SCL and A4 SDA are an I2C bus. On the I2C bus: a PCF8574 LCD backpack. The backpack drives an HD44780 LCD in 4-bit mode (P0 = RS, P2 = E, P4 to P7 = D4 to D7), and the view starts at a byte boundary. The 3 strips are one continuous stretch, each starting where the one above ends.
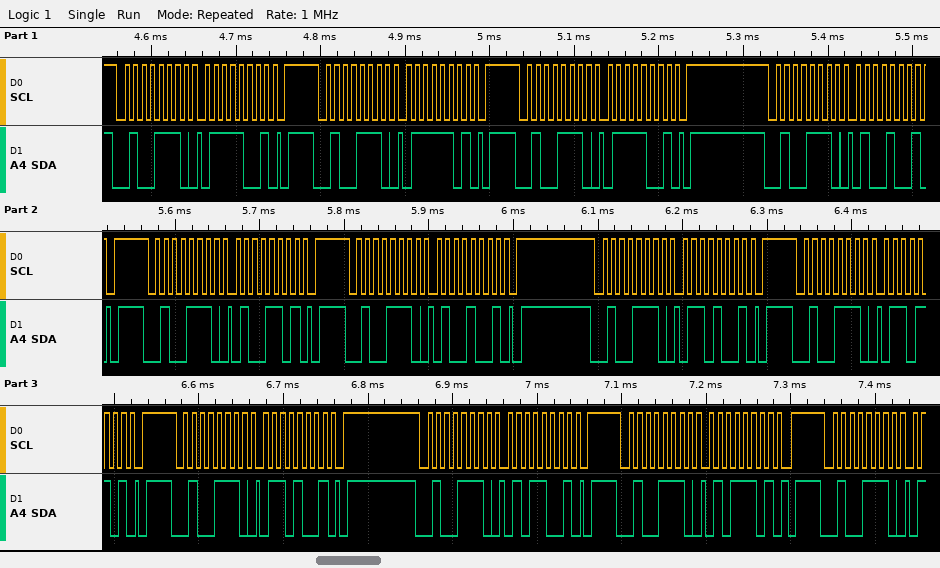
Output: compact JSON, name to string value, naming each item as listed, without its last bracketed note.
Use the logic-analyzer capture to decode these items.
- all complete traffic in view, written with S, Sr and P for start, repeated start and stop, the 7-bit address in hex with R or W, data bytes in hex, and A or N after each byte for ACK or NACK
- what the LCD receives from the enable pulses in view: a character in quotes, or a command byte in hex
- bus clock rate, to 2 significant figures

{"all complete traffic in view, written with S, Sr and P for start, repeated start and stop, the 7-bit address in hex with R or W, data bytes in hex, and A or N after each byte for ACK or NACK": "S 27W A 79 A P S 27W A 7D A P S 27W A 79 A P S 27W A 49 A P S 27W A 4D A P S 27W A 49 A P S 27W A 69 A P S 27W A 6D A P S 27W A 69 A P S 27W A 59 A P S 27W A 5D A P S 27W A", "what the LCD receives from the enable pulses in view: a character in quotes, or a command byte in hex": "'t'", "bus clock rate, to 2 significant figures": "100 kHz"}
